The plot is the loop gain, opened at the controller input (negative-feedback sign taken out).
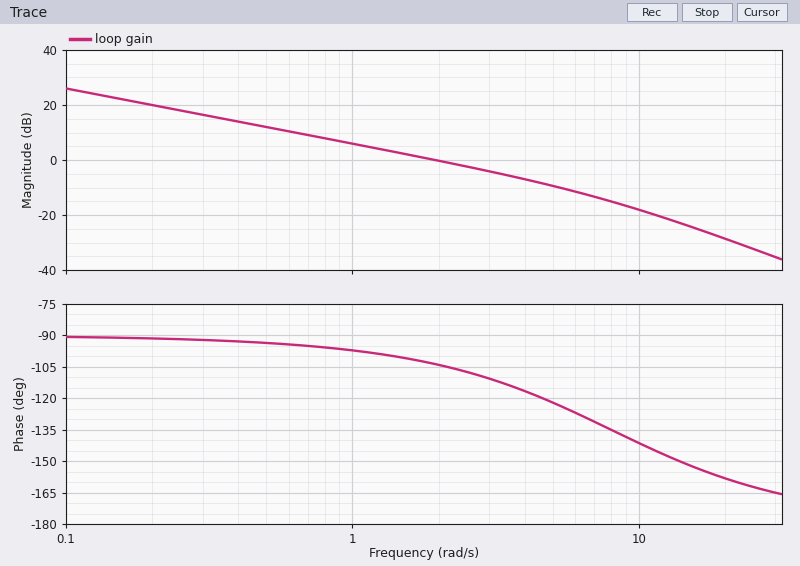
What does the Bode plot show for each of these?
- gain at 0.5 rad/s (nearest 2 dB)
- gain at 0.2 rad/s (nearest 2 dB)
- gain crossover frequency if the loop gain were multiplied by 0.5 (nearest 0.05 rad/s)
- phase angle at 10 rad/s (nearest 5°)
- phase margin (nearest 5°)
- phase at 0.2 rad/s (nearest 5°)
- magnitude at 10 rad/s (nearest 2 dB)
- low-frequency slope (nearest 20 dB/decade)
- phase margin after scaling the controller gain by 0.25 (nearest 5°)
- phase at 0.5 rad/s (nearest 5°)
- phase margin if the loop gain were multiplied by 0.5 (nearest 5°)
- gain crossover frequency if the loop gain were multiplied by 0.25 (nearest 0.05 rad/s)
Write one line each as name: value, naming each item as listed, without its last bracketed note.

gain at 0.5 rad/s: 12 dB
gain at 0.2 rad/s: 20 dB
gain crossover frequency if the loop gain were multiplied by 0.5: 1.00 rad/s
phase angle at 10 rad/s: -140°
phase margin: 75°
phase at 0.2 rad/s: -90°
magnitude at 10 rad/s: -18 dB
low-frequency slope: -20 dB/decade
phase margin after scaling the controller gain by 0.25: 85°
phase at 0.5 rad/s: -95°
phase margin if the loop gain were multiplied by 0.5: 85°
gain crossover frequency if the loop gain were multiplied by 0.25: 0.50 rad/s
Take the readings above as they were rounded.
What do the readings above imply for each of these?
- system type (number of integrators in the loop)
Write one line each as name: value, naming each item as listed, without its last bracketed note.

system type: 1
